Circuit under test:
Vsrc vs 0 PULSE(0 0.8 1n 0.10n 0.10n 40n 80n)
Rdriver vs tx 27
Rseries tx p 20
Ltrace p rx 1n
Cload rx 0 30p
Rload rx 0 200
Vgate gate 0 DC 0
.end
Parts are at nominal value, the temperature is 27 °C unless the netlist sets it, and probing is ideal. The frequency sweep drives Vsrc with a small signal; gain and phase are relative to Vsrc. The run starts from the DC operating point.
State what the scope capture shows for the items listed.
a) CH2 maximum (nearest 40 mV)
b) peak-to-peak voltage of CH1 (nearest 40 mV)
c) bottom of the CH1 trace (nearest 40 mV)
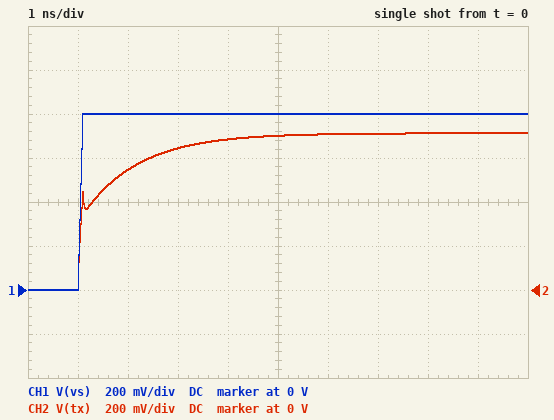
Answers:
720 mV
800 mV
0 V
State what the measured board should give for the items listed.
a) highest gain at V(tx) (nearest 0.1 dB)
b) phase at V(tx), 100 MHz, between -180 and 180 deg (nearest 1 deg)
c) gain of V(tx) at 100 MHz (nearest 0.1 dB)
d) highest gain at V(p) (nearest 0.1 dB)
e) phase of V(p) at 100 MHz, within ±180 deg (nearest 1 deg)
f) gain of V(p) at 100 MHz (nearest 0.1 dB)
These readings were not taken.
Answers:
-1.0 dB
-17 deg
-2.4 dB
-1.8 dB
-36 deg
-3.7 dB
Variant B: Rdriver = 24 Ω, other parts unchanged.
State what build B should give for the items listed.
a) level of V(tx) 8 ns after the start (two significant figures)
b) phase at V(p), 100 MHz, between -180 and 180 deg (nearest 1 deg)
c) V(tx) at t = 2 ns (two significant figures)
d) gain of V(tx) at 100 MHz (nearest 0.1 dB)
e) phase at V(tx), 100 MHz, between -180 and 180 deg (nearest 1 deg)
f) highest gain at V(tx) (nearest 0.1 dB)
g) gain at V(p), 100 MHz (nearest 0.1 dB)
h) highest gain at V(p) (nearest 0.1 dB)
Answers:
720 mV
-34 deg
570 mV
-2.1 dB
-15 deg
-0.9 dB
-3.4 dB
-1.7 dB
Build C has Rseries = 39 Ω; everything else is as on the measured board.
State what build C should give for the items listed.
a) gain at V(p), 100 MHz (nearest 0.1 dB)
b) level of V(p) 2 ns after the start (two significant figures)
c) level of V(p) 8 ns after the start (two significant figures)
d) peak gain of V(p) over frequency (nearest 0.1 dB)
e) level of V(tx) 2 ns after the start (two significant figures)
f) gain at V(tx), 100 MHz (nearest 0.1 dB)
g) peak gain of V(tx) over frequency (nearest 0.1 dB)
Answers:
-5.3 dB
280 mV
600 mV
-2.5 dB
590 mV
-2.3 dB
-0.9 dB
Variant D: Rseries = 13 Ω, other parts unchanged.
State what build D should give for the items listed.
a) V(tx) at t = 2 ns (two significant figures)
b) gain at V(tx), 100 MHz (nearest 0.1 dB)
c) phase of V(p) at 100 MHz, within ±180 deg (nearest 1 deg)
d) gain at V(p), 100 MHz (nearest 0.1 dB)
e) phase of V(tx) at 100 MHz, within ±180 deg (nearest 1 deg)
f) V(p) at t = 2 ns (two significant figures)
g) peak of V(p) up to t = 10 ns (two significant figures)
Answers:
530 mV
-2.3 dB
-32 deg
-3.1 dB
-19 deg
400 mV
670 mV
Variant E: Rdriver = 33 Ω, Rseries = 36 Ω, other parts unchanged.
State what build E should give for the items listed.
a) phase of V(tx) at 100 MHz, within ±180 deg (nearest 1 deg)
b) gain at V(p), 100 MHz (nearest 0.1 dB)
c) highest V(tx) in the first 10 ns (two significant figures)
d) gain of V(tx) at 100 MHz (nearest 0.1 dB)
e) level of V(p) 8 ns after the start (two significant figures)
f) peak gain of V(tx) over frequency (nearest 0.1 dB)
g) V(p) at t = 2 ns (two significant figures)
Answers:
-14 deg
-5.5 dB
700 mV
-2.8 dB
590 mV
-1.1 dB
270 mV
